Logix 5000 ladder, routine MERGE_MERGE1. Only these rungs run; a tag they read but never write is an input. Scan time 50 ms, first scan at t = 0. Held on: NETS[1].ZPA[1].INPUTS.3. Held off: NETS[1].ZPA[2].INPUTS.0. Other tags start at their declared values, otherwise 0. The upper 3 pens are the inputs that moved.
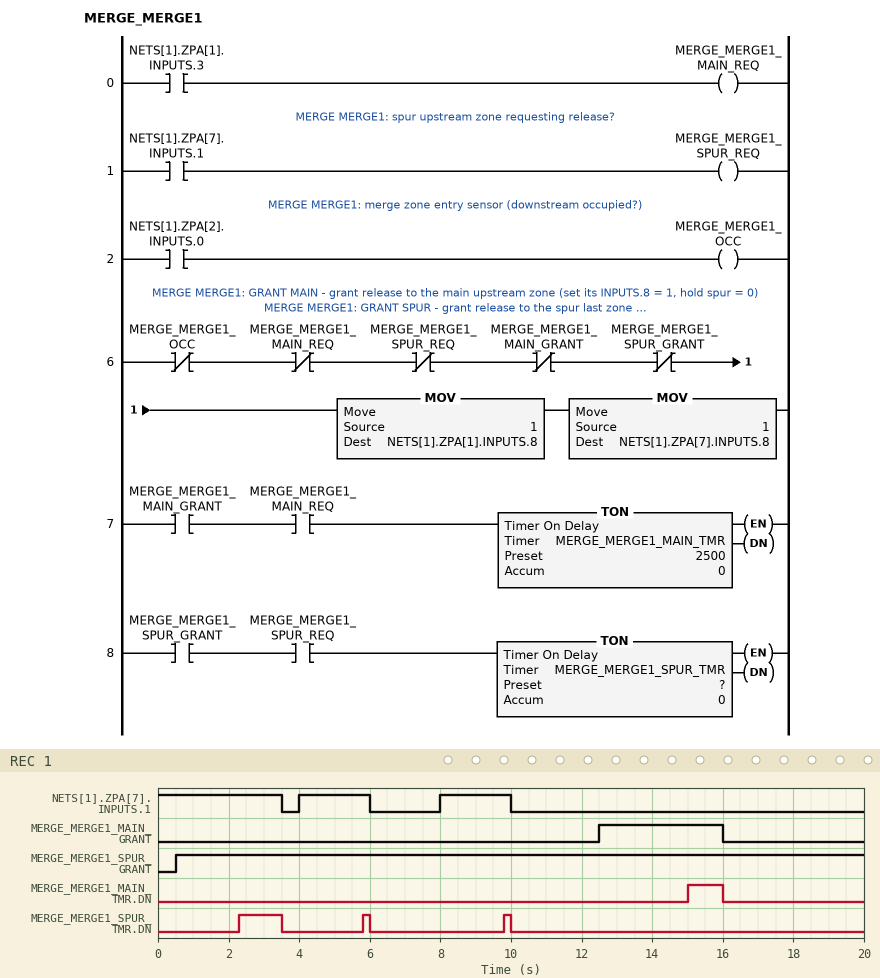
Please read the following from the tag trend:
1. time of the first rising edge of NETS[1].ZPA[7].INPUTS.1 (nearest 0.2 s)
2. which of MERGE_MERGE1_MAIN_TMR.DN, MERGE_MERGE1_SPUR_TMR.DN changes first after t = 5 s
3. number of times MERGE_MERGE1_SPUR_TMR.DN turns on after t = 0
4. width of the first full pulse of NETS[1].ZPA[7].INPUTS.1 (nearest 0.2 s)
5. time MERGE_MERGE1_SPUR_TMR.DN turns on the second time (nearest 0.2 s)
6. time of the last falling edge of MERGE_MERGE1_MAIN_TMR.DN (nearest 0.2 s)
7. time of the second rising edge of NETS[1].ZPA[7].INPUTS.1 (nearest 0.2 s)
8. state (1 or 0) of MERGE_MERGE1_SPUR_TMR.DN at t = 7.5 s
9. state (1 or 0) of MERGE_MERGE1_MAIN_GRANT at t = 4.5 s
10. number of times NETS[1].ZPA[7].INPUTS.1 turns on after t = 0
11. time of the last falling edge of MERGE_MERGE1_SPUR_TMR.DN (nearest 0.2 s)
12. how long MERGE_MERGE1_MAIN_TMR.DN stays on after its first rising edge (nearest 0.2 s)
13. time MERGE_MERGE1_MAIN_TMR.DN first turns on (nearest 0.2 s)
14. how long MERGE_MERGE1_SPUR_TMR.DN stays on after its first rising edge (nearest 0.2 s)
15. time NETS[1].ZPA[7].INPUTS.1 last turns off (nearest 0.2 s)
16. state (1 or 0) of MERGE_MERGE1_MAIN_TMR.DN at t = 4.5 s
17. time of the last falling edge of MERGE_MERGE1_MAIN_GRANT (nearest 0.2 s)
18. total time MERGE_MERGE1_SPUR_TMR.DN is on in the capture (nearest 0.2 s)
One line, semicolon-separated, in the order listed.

4.0 s; MERGE_MERGE1_SPUR_TMR.DN; 3; 2.0 s; 5.8 s; 16.0 s; 8.0 s; 0; 0; 2; 10.0 s; 1.0 s; 15.0 s; 1.2 s; 10.0 s; 0; 16.0 s; 1.6 s
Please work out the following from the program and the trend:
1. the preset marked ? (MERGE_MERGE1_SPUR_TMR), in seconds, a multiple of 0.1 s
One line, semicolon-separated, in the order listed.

1.8 s
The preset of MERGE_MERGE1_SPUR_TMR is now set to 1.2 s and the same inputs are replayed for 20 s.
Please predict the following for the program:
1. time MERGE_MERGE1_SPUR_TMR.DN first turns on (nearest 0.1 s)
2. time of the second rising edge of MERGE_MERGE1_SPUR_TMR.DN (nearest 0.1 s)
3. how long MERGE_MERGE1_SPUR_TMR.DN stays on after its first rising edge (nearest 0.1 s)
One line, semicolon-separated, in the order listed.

1.7 s; 5.2 s; 1.8 s
